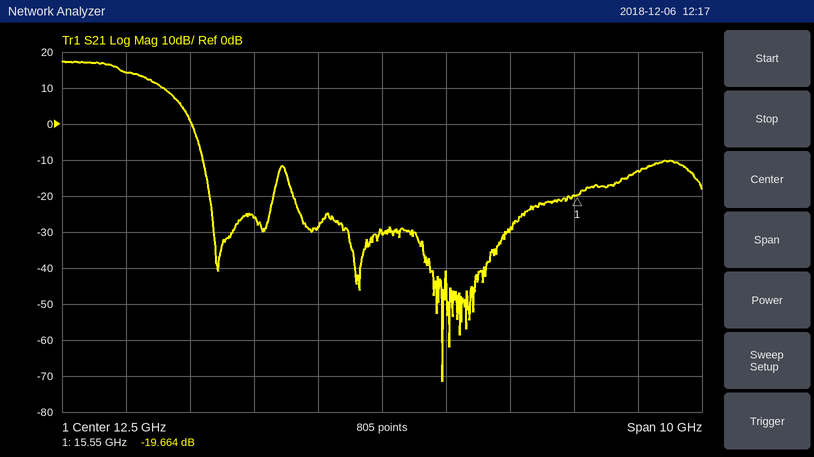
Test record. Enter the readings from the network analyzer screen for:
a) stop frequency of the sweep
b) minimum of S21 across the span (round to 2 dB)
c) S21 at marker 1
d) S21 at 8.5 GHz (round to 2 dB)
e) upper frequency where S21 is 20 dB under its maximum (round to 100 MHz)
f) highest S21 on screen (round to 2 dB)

17.5 GHz
-72 dB
-19.664 dB
14 dB
9.6 GHz
18 dB
